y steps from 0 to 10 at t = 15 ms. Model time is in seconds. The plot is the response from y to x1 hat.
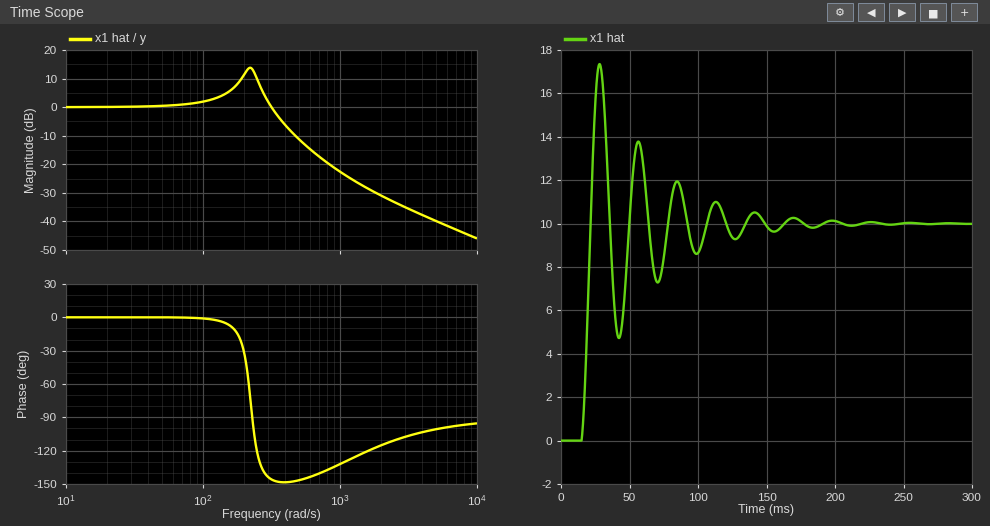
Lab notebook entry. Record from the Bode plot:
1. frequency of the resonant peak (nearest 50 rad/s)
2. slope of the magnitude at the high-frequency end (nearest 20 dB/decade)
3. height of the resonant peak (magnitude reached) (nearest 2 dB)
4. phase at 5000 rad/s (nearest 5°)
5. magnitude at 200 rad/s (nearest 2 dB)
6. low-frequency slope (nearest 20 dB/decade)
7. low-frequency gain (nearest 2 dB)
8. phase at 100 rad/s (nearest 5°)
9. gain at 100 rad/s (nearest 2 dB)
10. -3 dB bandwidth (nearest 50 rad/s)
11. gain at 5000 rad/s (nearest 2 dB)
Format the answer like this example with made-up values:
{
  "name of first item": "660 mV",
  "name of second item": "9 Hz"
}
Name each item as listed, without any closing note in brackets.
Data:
{
  "frequency of the resonant peak": "200 rad/s",
  "slope of the magnitude at the high-frequency end": "-20 dB/decade",
  "height of the resonant peak (magnitude reached)": "14 dB",
  "phase at 5000 rad/s": "-100°",
  "magnitude at 200 rad/s": "12 dB",
  "low-frequency slope": "0 dB/decade",
  "low-frequency gain": "0 dB",
  "phase at 100 rad/s": "0°",
  "gain at 100 rad/s": "2 dB",
  "-3 dB bandwidth": "350 rad/s",
  "gain at 5000 rad/s": "-40 dB"
}
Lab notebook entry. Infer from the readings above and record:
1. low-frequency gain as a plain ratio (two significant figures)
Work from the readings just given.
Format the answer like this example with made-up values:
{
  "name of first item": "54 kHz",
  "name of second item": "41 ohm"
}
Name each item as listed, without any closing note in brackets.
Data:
{
  "low-frequency gain as a plain ratio": "1.0"
}
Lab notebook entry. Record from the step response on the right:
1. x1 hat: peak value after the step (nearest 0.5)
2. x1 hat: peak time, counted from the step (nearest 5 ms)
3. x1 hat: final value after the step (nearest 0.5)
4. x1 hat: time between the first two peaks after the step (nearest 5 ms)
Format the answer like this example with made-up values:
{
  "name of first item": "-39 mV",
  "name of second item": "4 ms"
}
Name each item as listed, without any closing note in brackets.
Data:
{
  "x1 hat: peak value after the step": "17.5",
  "x1 hat: peak time, counted from the step": "15 ms",
  "x1 hat: final value after the step": "10.0",
  "x1 hat: time between the first two peaks after the step": "30 ms"
}
